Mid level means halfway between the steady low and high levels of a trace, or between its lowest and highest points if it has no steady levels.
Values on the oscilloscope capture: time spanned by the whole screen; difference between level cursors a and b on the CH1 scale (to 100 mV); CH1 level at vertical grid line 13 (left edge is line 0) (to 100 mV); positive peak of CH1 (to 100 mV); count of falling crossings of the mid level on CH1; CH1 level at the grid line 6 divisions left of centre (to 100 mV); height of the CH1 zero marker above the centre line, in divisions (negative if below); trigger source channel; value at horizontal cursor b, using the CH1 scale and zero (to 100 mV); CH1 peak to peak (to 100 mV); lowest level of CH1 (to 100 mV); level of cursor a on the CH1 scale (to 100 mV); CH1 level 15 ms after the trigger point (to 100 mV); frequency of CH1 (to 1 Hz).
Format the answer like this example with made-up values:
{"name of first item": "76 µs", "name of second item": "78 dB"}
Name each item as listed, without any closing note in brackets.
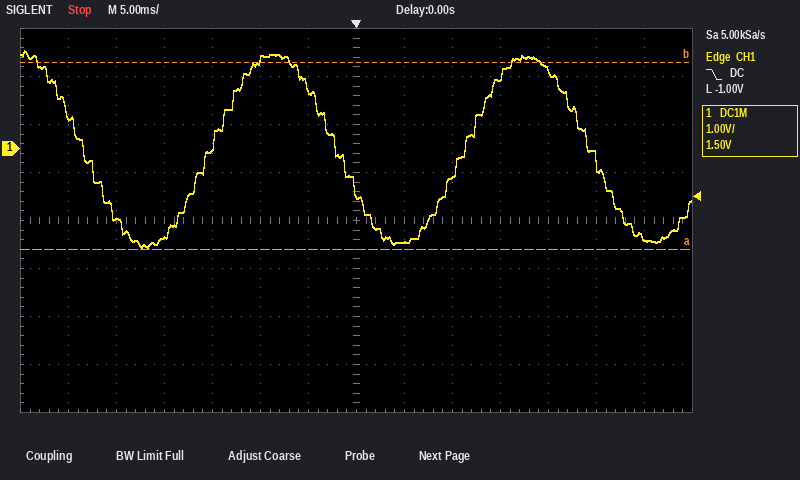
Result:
{"time spanned by the whole screen": "70 ms", "difference between level cursors a and b on the CH1 scale": "3.9 V", "CH1 level at vertical grid line 13 (left edge is line 0)": "-1.9 V", "positive peak of CH1": "2.0 V", "count of falling crossings of the mid level on CH1": "3", "CH1 level at the grid line 6 divisions left of centre": "700 mV", "height of the CH1 zero marker above the centre line, in divisions": "+1.5 div", "trigger source channel": "CH1", "value at horizontal cursor b, using the CH1 scale and zero": "1.8 V", "CH1 peak to peak": "4.1 V", "lowest level of CH1": "-2.1 V", "level of cursor a on the CH1 scale": "-2.1 V", "CH1 level 15 ms after the trigger point": "1.5 V", "frequency of CH1": "38 Hz"}
